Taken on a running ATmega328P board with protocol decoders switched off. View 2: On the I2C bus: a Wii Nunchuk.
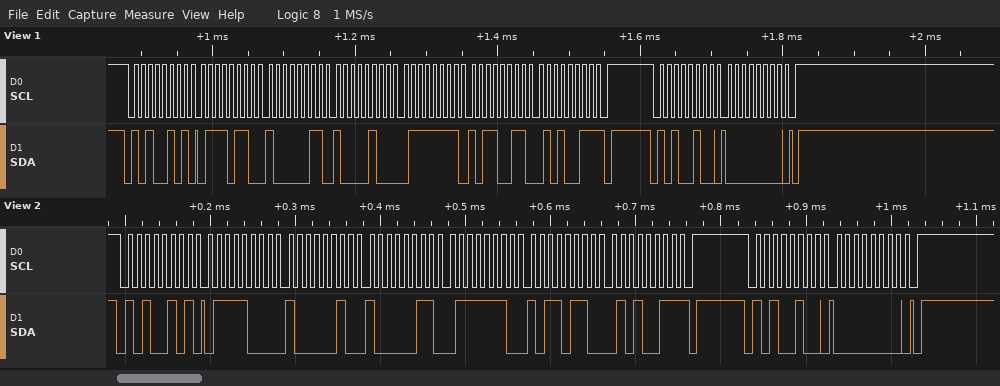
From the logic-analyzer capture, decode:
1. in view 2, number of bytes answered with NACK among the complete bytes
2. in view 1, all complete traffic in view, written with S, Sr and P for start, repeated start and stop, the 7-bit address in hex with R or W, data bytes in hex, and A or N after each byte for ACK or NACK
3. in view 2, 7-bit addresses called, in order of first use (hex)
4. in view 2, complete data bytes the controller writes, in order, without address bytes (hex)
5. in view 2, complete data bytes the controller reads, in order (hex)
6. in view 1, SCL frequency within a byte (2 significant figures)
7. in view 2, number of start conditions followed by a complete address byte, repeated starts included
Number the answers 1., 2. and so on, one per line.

1. 1
2. S 52R A 76 A 83 A 84 A 7F A B3 A 53 N P S 52W A 00 A P
3. 0x52
4. 00
5. 78 82 83 7E B6 53
6. 100 kHz
7. 2
